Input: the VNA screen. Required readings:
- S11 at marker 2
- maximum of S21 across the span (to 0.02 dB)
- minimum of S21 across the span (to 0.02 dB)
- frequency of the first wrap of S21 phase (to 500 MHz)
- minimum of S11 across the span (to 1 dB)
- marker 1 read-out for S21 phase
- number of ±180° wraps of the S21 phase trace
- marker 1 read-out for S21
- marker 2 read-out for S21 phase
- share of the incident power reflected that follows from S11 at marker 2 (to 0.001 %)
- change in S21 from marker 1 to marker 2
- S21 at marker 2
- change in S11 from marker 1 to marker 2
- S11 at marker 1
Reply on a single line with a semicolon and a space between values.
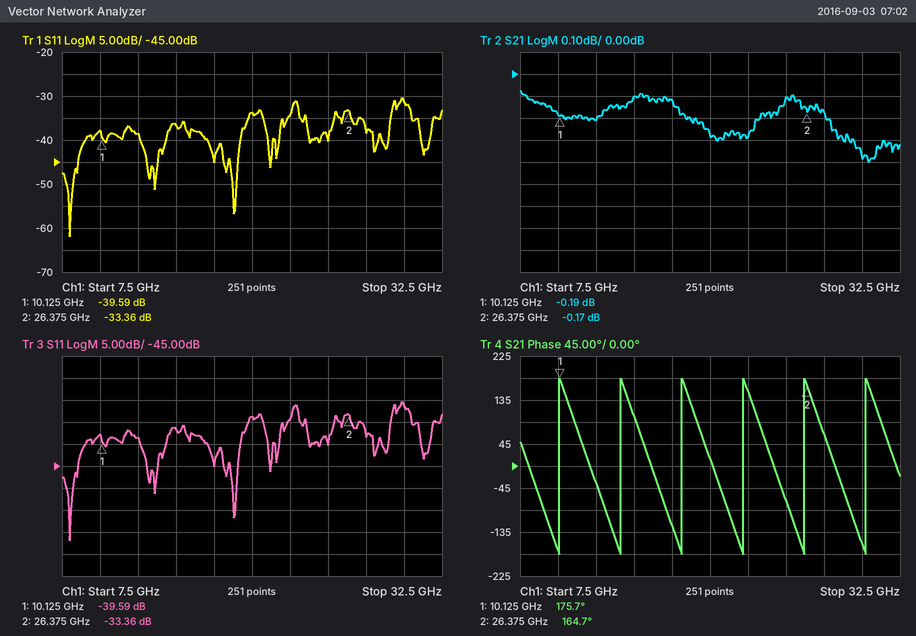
-33.36 dB; -0.08 dB; -0.40 dB; 10.0 GHz; -62 dB; 175.7°; 6; -0.19 dB; 164.7°; 0.046 %; 0.02 dB; -0.17 dB; 6.23 dB; -39.59 dB
